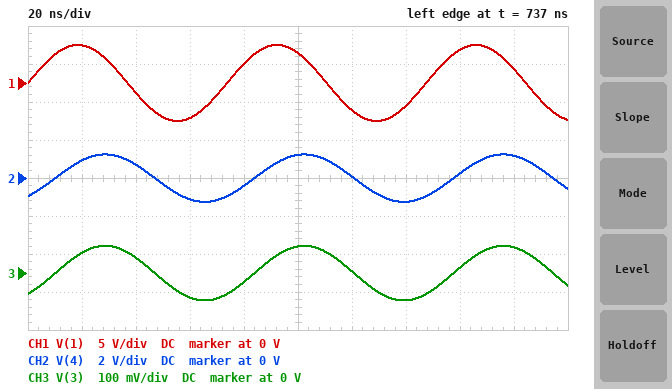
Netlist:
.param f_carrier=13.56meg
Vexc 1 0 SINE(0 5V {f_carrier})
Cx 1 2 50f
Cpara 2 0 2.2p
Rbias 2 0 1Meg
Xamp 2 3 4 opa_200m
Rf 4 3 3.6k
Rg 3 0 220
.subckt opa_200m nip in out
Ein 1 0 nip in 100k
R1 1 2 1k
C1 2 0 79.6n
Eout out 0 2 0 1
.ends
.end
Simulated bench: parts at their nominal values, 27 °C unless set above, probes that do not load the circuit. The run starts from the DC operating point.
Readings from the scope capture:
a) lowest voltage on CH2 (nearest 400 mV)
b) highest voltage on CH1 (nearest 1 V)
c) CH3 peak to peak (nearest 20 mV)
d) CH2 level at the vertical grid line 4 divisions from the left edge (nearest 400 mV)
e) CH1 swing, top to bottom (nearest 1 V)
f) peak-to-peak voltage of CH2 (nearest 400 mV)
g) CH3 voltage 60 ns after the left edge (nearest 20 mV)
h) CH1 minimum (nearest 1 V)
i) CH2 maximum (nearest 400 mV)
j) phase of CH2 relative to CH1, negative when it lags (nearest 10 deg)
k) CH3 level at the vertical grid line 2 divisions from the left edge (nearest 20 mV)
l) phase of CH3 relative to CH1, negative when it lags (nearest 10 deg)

-1.2 V
5 V
140 mV
-400 mV
10 V
2.4 V
-60 mV
-5 V
1.2 V
-50 deg
40 mV
-50 deg
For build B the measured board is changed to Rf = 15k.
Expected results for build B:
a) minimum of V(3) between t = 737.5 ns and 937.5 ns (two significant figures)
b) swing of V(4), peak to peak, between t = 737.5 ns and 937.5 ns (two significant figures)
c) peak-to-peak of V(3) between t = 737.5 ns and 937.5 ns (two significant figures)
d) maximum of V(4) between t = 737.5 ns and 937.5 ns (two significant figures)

-24 mV
3.2 V
46 mV
1.6 V
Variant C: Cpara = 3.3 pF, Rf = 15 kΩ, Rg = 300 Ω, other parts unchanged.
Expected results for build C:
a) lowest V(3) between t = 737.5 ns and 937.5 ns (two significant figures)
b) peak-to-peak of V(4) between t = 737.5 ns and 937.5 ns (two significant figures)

-21 mV
2.1 V
